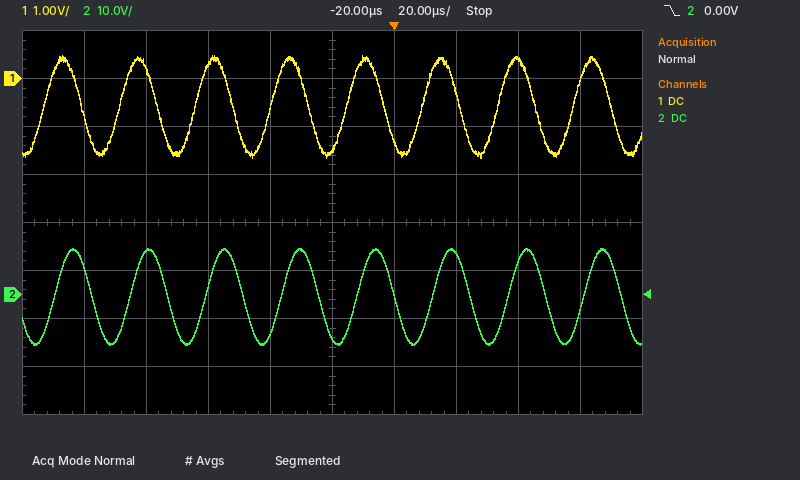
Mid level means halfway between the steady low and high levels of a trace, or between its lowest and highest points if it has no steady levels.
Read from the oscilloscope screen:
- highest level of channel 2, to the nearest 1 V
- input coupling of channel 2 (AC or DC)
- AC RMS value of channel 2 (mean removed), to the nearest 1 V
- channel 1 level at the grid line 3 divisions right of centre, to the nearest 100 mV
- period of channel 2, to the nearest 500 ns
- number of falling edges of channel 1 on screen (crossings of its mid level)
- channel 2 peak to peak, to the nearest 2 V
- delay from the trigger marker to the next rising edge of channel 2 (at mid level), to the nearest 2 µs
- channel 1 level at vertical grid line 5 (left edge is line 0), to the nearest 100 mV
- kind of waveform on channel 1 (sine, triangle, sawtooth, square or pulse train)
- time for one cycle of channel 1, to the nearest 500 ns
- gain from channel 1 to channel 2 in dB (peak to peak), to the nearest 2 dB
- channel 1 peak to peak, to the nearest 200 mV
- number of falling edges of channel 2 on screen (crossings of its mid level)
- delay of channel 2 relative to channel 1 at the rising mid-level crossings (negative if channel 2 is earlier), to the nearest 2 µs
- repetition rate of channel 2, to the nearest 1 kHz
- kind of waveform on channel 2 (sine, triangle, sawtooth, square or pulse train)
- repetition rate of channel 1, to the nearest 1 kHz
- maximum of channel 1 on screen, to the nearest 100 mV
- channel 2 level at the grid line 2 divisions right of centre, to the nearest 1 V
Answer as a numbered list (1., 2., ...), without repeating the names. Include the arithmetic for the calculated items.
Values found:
1. 10 V
2. DC
3. 20 V / (2√2) ≈ 7 V
4. 400 mV
5. 24.5 µs
6. 8
7. 20 V
8. 12 µs
9. -1.5 V
10. sine
11. 24.5 µs
12. 20 log10(20 V / 2.2 V) ≈ 19.2 dB, so 20 dB to the nearest 2 dB
13. 2.2 V
14. 8
15. +4 µs
16. 1 / 24.5 µs ≈ 41 kHz
17. sine
18. 1 / 24.5 µs ≈ 41 kHz
19. 500 mV
20. 8 V
